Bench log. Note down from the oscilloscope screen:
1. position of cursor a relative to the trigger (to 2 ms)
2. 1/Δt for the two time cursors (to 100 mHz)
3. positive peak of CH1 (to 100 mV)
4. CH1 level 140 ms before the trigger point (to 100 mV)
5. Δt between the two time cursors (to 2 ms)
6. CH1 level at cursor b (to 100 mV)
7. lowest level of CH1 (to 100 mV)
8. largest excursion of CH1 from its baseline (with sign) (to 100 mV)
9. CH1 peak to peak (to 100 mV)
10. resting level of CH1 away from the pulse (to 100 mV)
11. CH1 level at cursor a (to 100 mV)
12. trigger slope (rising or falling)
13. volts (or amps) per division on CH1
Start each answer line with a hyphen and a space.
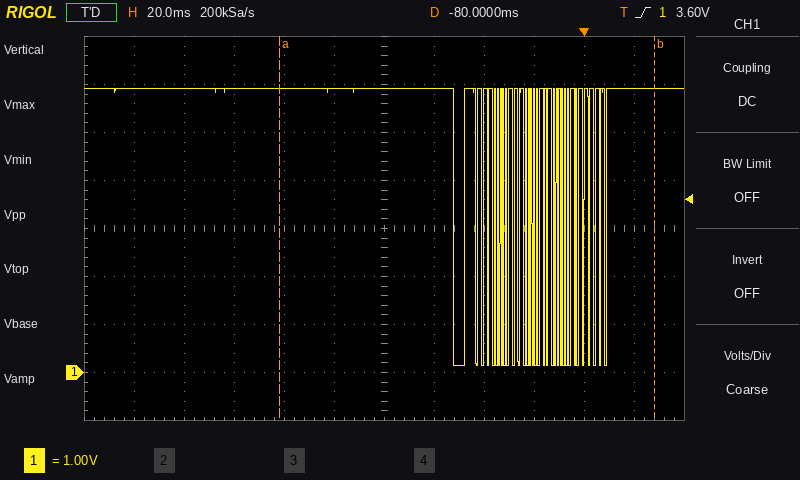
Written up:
- -122 ms
- 6.7 Hz
- 5.9 V
- 5.9 V
- 150 ms
- 5.9 V
- 100 mV
- -5.8 V
- 5.8 V
- 5.9 V
- 5.9 V
- rising
- 1 V
